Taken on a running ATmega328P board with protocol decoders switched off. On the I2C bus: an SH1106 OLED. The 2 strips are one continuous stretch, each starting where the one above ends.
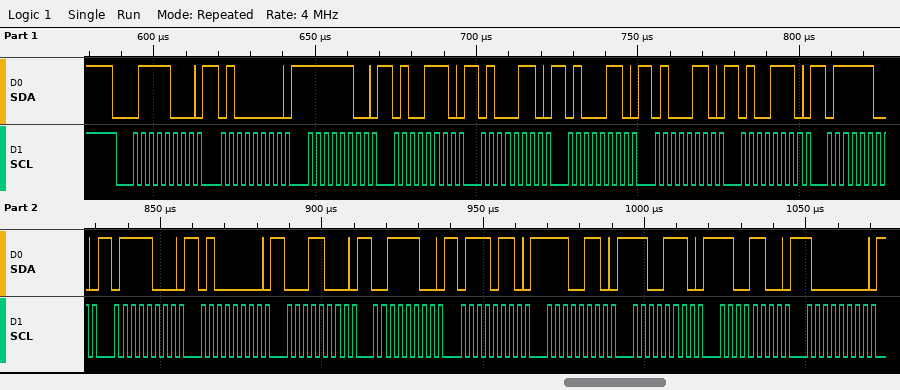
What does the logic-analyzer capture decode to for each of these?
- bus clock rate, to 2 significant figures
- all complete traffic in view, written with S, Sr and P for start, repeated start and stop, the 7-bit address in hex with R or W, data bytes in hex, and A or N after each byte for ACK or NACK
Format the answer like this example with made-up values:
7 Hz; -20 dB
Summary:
400 kHz; S 3CW A 40 A FC A 4E A 46 A 46 A 46 A 4E A 7C A 78 A 40 A 18 A 3C A 76 A E6 A CE A CC A 80 A
